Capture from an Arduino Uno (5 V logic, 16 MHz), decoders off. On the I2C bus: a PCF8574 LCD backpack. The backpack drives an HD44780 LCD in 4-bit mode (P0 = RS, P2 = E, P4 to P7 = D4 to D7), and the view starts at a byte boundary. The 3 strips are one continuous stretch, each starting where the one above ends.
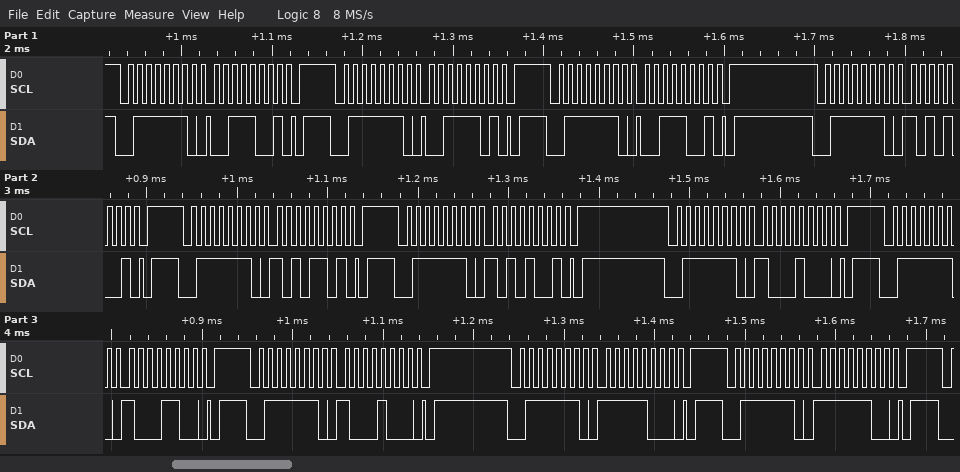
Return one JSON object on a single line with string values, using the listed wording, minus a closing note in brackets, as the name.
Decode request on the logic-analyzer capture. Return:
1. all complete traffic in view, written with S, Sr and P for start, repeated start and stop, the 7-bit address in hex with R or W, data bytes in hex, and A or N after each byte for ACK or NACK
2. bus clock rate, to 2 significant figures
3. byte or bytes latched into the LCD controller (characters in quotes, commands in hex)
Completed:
{"all complete traffic in view, written with S, Sr and P for start, repeated start and stop, the 7-bit address in hex with R or W, data bytes in hex, and A or N after each byte for ACK or NACK": "S 3FW A 39 A P S 3FW A 3D A P S 3FW A 39 A P S 3FW A A9 A P S 3FW A AD A P S 3FW A A9 A P S 3FW A 88 A P S 3FW A 8C A P S 3FW A 88 A P S 3FW A F8 A P S 3FW A FC A P", "bus clock rate, to 2 significant figures": "100 kHz", "byte or bytes latched into the LCD controller": "':'"}
